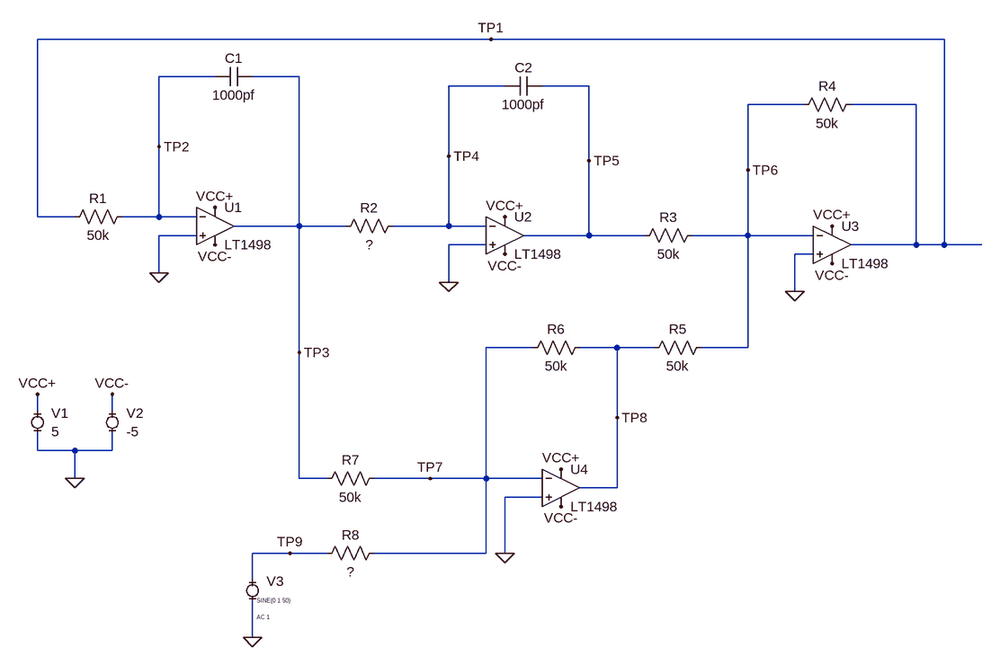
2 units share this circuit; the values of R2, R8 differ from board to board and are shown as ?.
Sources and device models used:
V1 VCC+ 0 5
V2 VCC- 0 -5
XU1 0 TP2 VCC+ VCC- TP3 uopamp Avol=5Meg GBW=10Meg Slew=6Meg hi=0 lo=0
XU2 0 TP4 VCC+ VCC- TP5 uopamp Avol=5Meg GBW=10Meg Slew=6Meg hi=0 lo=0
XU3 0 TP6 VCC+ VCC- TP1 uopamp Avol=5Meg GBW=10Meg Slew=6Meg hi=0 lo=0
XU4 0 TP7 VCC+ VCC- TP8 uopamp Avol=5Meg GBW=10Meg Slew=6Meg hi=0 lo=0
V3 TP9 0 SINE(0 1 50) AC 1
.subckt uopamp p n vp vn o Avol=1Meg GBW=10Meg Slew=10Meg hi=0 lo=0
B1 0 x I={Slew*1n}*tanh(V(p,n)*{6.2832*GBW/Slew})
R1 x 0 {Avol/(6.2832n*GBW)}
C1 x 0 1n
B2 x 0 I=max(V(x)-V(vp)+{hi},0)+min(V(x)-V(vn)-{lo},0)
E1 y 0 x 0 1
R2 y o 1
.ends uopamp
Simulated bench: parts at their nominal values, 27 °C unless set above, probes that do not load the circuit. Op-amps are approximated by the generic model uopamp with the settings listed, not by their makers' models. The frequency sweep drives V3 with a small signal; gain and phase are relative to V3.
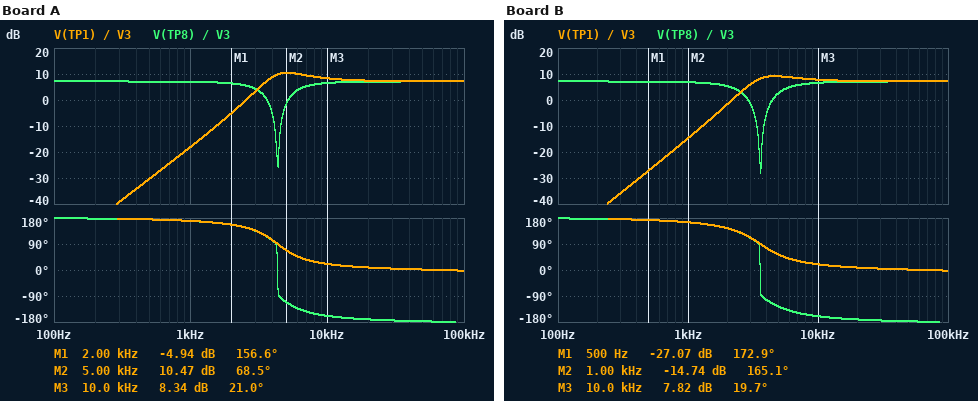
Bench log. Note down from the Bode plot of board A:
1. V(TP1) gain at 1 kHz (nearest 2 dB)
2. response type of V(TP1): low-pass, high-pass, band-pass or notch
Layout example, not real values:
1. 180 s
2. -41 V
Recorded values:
1. -18 dB
2. high-pass
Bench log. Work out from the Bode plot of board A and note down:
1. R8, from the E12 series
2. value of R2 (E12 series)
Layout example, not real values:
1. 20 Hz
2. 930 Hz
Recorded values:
1. 22 kΩ
2. 27 kΩ
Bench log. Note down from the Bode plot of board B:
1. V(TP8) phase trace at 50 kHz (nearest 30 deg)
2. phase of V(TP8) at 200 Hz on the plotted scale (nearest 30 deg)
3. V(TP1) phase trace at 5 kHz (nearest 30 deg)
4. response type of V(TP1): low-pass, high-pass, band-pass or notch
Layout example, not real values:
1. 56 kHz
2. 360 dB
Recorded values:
1. -180 deg
2. 180 deg
3. 60 deg
4. high-pass
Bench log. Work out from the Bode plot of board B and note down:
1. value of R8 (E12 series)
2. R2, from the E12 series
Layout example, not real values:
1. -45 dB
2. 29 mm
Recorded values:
1. 22 kΩ
2. 39 kΩ
